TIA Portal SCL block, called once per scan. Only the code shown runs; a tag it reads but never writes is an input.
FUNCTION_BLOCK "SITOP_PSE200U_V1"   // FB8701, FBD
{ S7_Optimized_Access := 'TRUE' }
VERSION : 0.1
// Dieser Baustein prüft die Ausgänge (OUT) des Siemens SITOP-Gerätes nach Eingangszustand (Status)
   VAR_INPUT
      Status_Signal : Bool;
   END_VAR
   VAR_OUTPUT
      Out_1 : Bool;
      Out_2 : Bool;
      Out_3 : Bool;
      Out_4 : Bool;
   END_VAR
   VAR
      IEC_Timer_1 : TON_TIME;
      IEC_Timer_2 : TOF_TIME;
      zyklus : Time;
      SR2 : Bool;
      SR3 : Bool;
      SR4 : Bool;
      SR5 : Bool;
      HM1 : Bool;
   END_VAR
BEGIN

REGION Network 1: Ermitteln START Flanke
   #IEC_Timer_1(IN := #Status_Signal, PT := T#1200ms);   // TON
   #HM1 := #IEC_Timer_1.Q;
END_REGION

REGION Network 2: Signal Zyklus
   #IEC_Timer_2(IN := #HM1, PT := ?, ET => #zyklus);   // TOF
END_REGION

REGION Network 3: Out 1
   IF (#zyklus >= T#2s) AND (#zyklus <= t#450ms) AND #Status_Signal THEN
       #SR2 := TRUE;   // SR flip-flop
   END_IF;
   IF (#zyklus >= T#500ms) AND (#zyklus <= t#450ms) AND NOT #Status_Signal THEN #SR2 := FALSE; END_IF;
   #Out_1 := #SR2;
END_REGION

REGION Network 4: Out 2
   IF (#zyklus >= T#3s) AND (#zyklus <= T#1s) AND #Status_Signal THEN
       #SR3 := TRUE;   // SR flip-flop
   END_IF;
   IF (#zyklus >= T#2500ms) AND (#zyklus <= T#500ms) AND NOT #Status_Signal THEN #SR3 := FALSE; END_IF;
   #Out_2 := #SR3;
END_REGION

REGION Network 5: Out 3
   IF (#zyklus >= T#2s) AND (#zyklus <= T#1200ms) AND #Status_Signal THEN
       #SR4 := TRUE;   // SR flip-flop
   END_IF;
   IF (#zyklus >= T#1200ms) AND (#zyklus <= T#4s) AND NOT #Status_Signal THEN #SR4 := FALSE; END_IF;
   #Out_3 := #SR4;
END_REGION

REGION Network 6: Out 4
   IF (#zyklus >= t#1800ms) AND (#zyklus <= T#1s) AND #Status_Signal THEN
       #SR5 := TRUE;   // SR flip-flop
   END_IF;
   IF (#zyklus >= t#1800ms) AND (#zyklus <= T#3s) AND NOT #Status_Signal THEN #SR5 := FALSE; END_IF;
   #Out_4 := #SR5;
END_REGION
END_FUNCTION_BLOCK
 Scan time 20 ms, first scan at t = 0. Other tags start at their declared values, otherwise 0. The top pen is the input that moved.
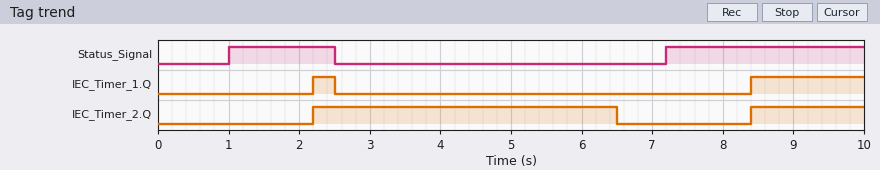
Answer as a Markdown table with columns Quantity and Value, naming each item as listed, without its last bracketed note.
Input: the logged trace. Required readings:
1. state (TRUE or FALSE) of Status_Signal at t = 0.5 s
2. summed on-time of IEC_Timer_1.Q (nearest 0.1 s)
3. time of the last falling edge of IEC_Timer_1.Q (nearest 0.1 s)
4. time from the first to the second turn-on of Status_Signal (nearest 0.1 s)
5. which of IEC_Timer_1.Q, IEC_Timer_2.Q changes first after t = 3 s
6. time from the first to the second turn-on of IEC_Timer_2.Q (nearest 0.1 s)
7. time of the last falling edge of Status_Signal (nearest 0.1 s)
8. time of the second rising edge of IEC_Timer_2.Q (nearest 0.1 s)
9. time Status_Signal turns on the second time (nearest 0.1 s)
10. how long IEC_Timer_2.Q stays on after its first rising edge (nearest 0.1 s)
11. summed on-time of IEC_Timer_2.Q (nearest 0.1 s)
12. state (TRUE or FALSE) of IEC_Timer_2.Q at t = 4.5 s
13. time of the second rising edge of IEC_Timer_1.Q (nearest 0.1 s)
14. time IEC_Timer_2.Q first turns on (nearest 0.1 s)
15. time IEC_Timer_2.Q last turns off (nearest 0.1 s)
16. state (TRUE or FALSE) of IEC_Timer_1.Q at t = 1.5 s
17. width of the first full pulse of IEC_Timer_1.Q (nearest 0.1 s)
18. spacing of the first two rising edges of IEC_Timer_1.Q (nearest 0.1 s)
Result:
| Quantity | Value |
|---|---|
| state (TRUE or FALSE) of Status_Signal at t = 0.5 s | FALSE |
| summed on-time of IEC_Timer_1.Q | 1.9 s |
| time of the last falling edge of IEC_Timer_1.Q | 2.5 s |
| time from the first to the second turn-on of Status_Signal | 6.2 s |
| which of IEC_Timer_1.Q, IEC_Timer_2.Q changes first after t = 3 s | IEC_Timer_2.Q |
| time from the first to the second turn-on of IEC_Timer_2.Q | 6.2 s |
| time of the last falling edge of Status_Signal | 2.5 s |
| time of the second rising edge of IEC_Timer_2.Q | 8.4 s |
| time Status_Signal turns on the second time | 7.2 s |
| how long IEC_Timer_2.Q stays on after its first rising edge | 4.3 s |
| summed on-time of IEC_Timer_2.Q | 5.9 s |
| state (TRUE or FALSE) of IEC_Timer_2.Q at t = 4.5 s | TRUE |
| time of the second rising edge of IEC_Timer_1.Q | 8.4 s |
| time IEC_Timer_2.Q first turns on | 2.2 s |
| time IEC_Timer_2.Q last turns off | 6.5 s |
| state (TRUE or FALSE) of IEC_Timer_1.Q at t = 1.5 s | FALSE |
| width of the first full pulse of IEC_Timer_1.Q | 0.3 s |
| spacing of the first two rising edges of IEC_Timer_1.Q | 6.2 s |
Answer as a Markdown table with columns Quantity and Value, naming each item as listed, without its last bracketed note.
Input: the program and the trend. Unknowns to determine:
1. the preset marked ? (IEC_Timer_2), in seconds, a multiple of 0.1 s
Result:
| Quantity | Value |
|---|---|
| the preset marked ? (IEC_Timer_2), in seconds, a multiple of 0.1 s | 4.0 s |
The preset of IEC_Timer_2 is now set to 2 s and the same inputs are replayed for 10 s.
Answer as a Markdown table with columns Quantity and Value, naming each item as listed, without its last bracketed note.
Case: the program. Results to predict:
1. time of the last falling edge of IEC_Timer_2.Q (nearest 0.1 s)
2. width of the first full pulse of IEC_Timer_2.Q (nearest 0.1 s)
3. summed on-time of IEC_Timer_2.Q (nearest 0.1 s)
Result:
| Quantity | Value |
|---|---|
| time of the last falling edge of IEC_Timer_2.Q | 4.5 s |
| width of the first full pulse of IEC_Timer_2.Q | 2.3 s |
| summed on-time of IEC_Timer_2.Q | 3.9 s |
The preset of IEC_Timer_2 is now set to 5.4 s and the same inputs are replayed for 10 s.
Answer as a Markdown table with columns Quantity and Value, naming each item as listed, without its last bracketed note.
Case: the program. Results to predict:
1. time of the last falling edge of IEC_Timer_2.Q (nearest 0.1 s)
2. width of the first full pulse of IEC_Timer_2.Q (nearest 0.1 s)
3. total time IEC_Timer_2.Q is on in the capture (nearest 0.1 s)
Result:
| Quantity | Value |
|---|---|
| time of the last falling edge of IEC_Timer_2.Q | 7.9 s |
| width of the first full pulse of IEC_Timer_2.Q | 5.7 s |
| total time IEC_Timer_2.Q is on in the capture | 7.3 s |
